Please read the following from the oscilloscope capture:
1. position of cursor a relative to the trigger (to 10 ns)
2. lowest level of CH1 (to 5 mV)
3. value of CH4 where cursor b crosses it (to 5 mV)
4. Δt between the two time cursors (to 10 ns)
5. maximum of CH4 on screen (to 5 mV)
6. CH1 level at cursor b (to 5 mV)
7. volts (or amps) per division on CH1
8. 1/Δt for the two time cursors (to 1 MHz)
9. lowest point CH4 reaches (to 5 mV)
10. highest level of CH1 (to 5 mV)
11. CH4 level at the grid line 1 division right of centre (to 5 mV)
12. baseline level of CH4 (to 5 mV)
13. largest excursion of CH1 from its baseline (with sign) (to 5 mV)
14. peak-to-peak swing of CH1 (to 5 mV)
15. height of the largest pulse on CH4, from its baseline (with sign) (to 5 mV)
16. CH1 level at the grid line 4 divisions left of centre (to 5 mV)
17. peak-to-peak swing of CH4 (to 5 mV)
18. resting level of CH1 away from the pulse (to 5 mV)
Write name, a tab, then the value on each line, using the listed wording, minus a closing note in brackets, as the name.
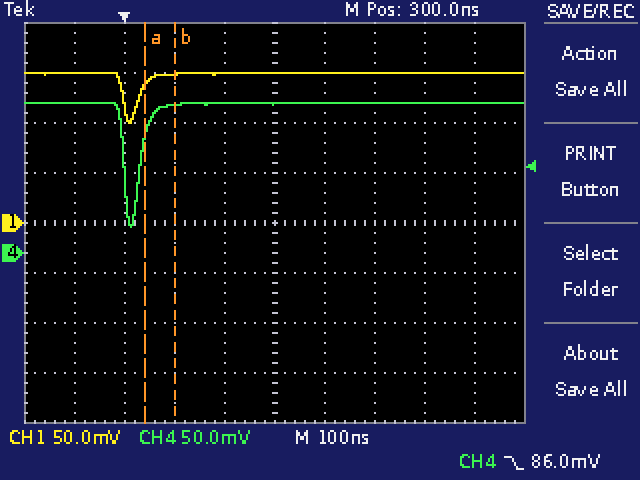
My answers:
position of cursor a relative to the trigger	+40 ns
lowest level of CH1	100 mV
value of CH4 where cursor b crosses it	150 mV
Δt between the two time cursors	60 ns
maximum of CH4 on screen	150 mV
CH1 level at cursor b	150 mV
volts (or amps) per division on CH1	50 mV
1/Δt for the two time cursors	17 MHz
lowest point CH4 reaches	25 mV
highest level of CH1	150 mV
CH4 level at the grid line 1 division right of centre	150 mV
baseline level of CH4	150 mV
largest excursion of CH1 from its baseline (with sign)	-50 mV
peak-to-peak swing of CH1	50 mV
height of the largest pulse on CH4, from its baseline (with sign)	-125 mV
CH1 level at the grid line 4 divisions left of centre	150 mV
peak-to-peak swing of CH4	125 mV
resting level of CH1 away from the pulse	150 mV
